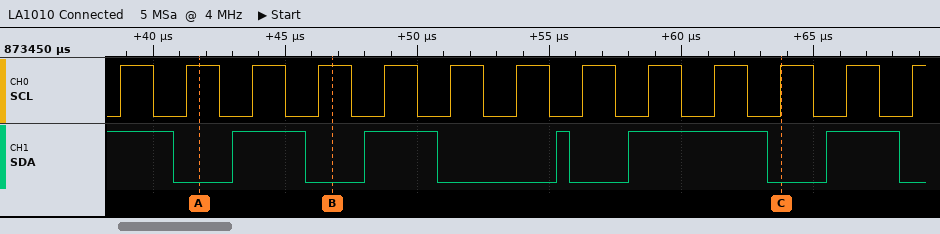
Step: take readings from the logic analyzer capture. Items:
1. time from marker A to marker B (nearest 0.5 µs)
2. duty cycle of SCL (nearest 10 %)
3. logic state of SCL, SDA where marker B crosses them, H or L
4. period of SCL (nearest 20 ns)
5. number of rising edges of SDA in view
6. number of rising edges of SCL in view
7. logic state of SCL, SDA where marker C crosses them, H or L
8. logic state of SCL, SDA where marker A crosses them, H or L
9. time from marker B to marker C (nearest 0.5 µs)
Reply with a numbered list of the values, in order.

1. 5 µs
2. 50 %
3. SCL=H, SDA=L
4. 2500 ns
5. 5
6. 13
7. SCL=H, SDA=L
8. SCL=H, SDA=L
9. 17 µs
